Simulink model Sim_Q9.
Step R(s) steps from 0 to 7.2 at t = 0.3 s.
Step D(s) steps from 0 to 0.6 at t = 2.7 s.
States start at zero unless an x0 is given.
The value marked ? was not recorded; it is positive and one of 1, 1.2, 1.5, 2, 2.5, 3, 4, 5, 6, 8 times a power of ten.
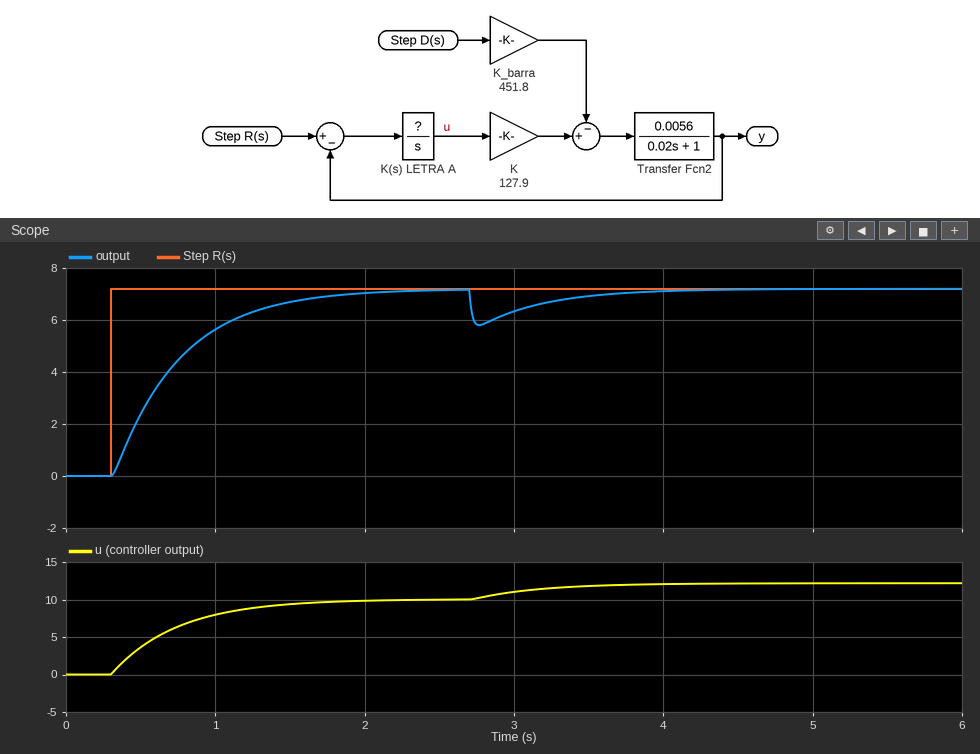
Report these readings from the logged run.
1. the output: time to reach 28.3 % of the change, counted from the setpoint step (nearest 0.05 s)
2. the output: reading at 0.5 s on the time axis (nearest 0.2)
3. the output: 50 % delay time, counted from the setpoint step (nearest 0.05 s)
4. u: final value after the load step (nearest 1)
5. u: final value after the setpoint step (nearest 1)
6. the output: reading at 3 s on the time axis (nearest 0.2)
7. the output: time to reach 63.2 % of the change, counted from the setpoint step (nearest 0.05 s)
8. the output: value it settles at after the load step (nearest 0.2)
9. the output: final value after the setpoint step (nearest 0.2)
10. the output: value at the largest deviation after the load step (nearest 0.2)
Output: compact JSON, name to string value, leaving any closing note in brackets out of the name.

{"the output: time to reach 28.3 % of the change, counted from the setpoint step": "0.15 s", "the output: reading at 0.5 s on the time axis": "2.4", "the output: 50 % delay time, counted from the setpoint step": "0.35 s", "u: final value after the load step": "12", "u: final value after the setpoint step": "10", "the output: reading at 3 s on the time axis": "6.4", "the output: time to reach 63.2 % of the change, counted from the setpoint step": "0.45 s", "the output: value it settles at after the load step": "7.2", "the output: final value after the setpoint step": "7.2", "the output: value at the largest deviation after the load step": "5.8"}
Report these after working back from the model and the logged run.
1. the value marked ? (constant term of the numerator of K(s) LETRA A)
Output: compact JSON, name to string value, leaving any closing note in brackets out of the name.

{"the value marked ? (constant term of the numerator of K(s) LETRA A)": "3"}
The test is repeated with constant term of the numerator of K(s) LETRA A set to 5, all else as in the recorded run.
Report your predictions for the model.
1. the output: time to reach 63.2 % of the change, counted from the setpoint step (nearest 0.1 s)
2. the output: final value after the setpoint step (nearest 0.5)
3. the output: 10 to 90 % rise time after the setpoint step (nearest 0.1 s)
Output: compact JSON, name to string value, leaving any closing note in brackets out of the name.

{"the output: time to reach 63.2 % of the change, counted from the setpoint step": "0.3 s", "the output: final value after the setpoint step": "7.0", "the output: 10 to 90 % rise time after the setpoint step": "0.6 s"}
